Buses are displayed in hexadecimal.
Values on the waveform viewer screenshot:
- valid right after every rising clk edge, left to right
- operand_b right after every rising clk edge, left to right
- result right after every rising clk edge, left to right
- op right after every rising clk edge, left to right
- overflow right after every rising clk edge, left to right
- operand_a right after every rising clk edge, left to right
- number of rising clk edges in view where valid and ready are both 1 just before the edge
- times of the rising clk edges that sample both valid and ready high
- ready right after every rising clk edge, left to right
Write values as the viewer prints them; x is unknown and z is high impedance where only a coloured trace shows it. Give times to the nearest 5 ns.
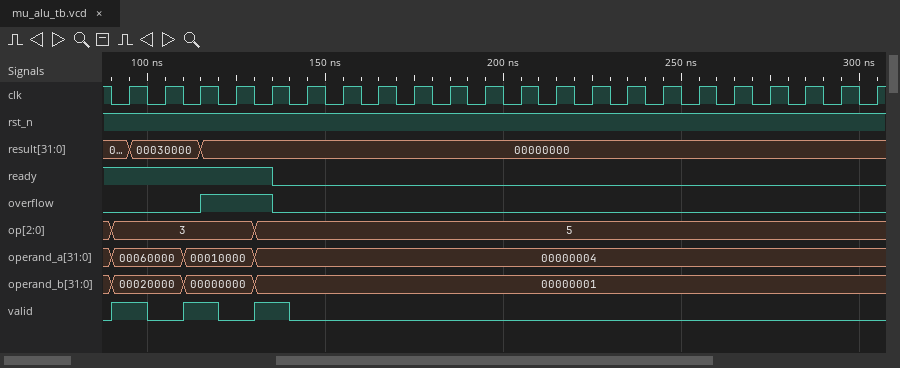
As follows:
1 0 1 0 1 0 0 0 0 0 0 0 0 0 0 0 0 0 0 0 0 0
00020000, 00020000, 00000000, 00000000, 00000001, 00000001, 00000001, 00000001, 00000001, 00000001, 00000001, 00000001, 00000001, 00000001, 00000001, 00000001, 00000001, 00000001, 00000001, 00000001, 00000001, 00000001
00030000, 00030000, 00000000, 00000000, 00000000, 00000000, 00000000, 00000000, 00000000, 00000000, 00000000, 00000000, 00000000, 00000000, 00000000, 00000000, 00000000, 00000000, 00000000, 00000000, 00000000, 00000000
3, 3, 3, 3, 5, 5, 5, 5, 5, 5, 5, 5, 5, 5, 5, 5, 5, 5, 5, 5, 5, 5
0 0 1 1 0 0 0 0 0 0 0 0 0 0 0 0 0 0 0 0 0 0
00060000, 00060000, 00010000, 00010000, 00000004, 00000004, 00000004, 00000004, 00000004, 00000004, 00000004, 00000004, 00000004, 00000004, 00000004, 00000004, 00000004, 00000004, 00000004, 00000004, 00000004, 00000004
3
95 ns, 115 ns, 135 ns
1 1 1 1 0 0 0 0 0 0 0 0 0 0 0 0 0 0 0 0 0 0
